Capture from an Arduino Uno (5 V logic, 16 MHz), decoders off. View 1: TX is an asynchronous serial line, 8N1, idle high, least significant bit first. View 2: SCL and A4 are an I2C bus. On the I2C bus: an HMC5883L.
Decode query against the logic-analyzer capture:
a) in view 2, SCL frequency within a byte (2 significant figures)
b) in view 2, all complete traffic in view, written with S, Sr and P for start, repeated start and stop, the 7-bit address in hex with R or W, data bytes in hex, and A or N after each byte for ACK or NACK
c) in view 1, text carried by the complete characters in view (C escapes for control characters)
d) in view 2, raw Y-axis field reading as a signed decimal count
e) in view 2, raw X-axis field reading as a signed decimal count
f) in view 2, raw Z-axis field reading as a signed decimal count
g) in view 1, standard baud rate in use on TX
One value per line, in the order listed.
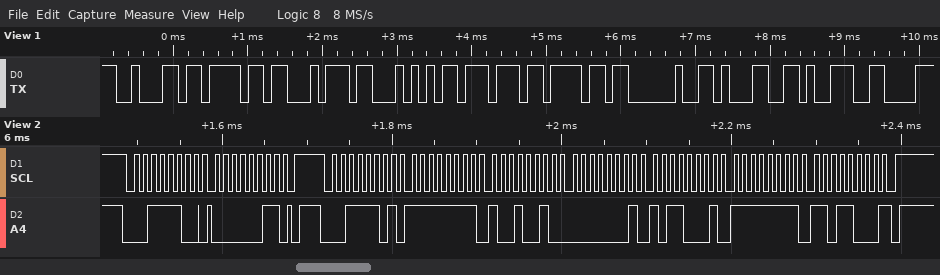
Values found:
100 kHz
S 1EW A 03 A P S 1ER A FF A 92 A 01 A B1 A FF A D8 N P
"botTwo 19"
-40
-110
433
9600 baud
